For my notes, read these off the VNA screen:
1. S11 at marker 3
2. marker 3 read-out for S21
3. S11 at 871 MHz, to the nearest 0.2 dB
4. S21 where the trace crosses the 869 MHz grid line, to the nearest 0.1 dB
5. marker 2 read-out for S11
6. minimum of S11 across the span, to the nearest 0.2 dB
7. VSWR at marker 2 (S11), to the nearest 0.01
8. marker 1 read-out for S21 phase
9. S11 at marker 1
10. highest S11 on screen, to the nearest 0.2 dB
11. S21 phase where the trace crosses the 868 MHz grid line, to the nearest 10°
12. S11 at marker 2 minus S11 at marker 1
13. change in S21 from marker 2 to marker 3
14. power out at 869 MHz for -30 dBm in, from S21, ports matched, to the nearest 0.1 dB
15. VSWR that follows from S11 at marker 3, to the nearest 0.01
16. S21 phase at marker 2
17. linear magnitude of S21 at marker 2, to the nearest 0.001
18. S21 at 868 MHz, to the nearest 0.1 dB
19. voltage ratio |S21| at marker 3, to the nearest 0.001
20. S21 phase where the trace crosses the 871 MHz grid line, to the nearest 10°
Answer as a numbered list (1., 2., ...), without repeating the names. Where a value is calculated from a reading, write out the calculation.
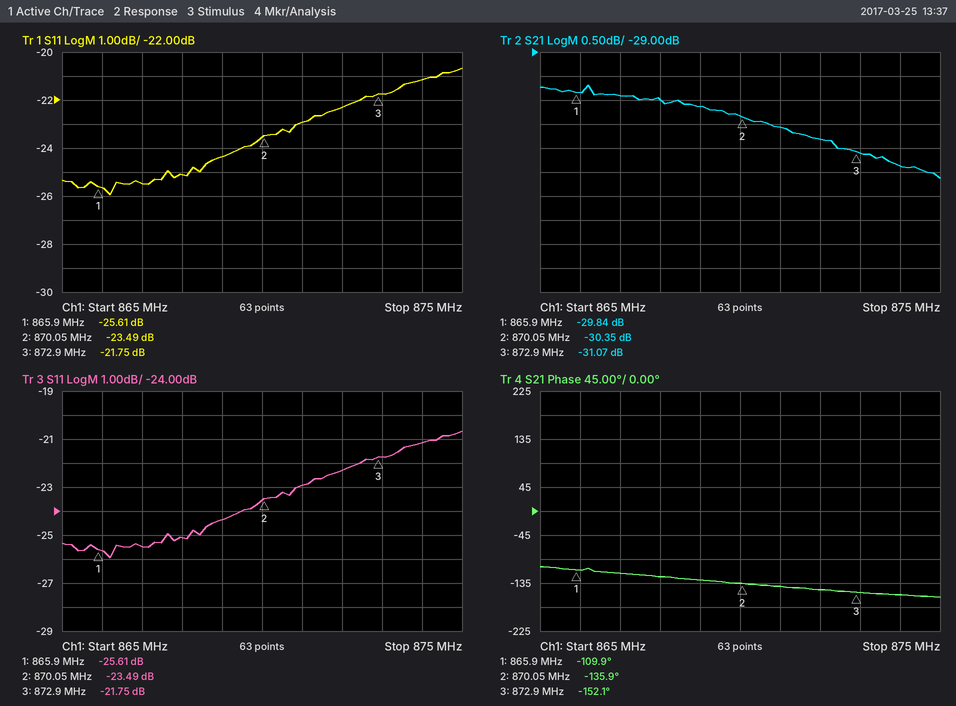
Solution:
1. -21.75 dB
2. -31.07 dB
3. -23.0 dB
4. -30.1 dB
5. -23.49 dB
6. -26.0 dB
7. (1 + 0.0669)/(1 − 0.0669) ≈ 1.14
8. -109.9°
9. -25.61 dB
10. -20.6 dB
11. -120°
12. -23.49 − (-25.61) = 2.12 dB
13. -31.07 − (-30.35) = -0.72 dB
14. -30 dBm + (-30.1 dB) = -60.1 dBm
15. (1 + 0.0818)/(1 − 0.0818) ≈ 1.18
16. -135.9°
17. 10^(-30.35/20) ≈ 0.030
18. -30.0 dB
19. 10^(-31.07/20) ≈ 0.028
20. -140°
